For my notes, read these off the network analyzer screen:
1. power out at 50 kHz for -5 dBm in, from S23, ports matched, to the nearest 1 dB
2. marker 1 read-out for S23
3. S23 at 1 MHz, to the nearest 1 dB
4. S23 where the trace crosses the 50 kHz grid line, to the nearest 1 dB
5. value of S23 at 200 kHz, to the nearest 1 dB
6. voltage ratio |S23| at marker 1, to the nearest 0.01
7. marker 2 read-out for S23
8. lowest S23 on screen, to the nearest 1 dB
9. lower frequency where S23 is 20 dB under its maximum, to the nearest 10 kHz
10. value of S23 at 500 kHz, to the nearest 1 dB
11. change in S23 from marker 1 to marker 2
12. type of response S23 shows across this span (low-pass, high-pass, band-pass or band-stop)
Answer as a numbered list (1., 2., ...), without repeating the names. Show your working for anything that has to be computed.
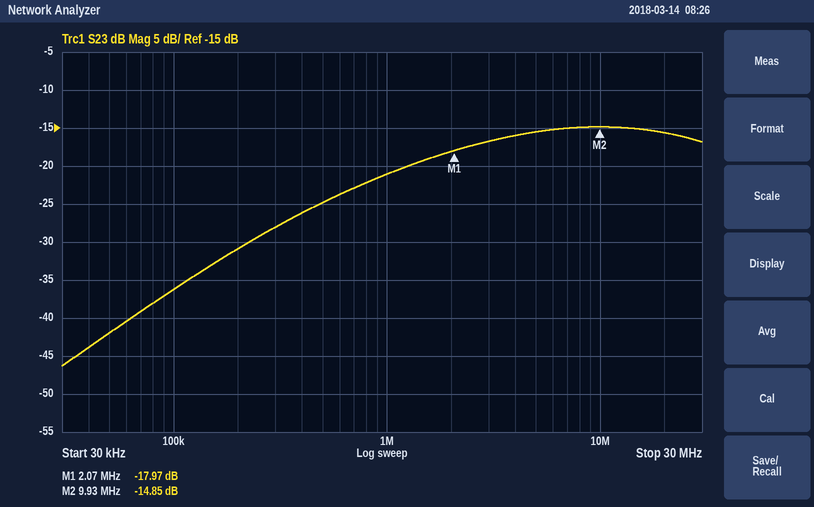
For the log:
1. -5 dBm + (-42 dB) = -47 dBm
2. -17.97 dB
3. -21 dB
4. -42 dB
5. -31 dB
6. 10^(-17.97/20) ≈ 0.13
7. -14.85 dB
8. -46 dB
9. 120 kHz
10. -25 dB
11. -14.85 − (-17.97) = 3.12 dB
12. high-pass
